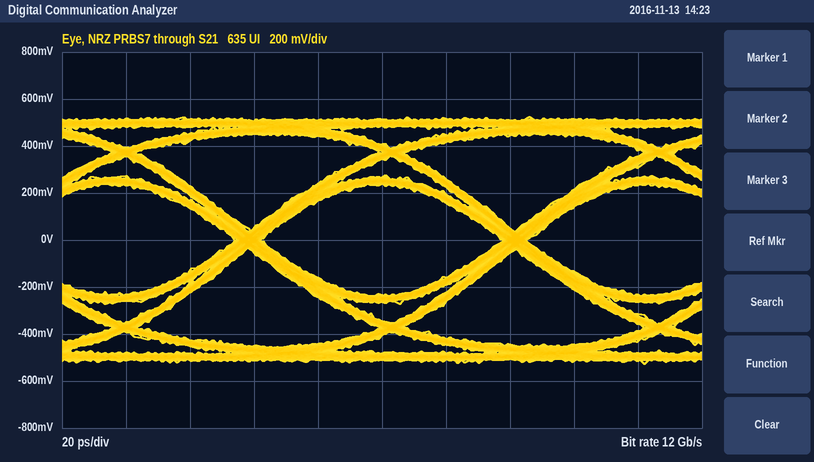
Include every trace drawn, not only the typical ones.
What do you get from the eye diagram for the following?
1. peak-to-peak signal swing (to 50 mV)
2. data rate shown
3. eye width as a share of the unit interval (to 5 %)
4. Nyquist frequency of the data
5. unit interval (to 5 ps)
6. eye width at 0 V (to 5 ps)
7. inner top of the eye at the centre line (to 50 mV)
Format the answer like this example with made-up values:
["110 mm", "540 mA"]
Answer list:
["1.05 V", "12 Gb/s", "90 %", "6 GHz", "85 ps", "75 ps", "250 mV"]
